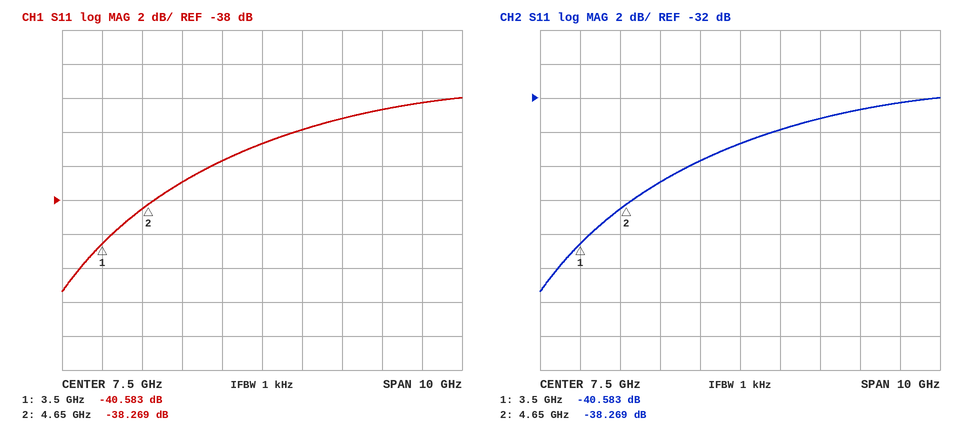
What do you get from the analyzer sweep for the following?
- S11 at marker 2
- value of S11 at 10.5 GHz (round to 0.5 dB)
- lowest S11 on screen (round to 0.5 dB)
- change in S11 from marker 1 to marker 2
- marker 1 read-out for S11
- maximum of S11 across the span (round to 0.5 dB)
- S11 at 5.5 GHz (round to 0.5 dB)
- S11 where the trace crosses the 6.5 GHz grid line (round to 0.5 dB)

-38.269 dB
-32.5 dB
-43.5 dB
2.314 dB
-40.583 dB
-32.0 dB
-37.0 dB
-35.5 dB
